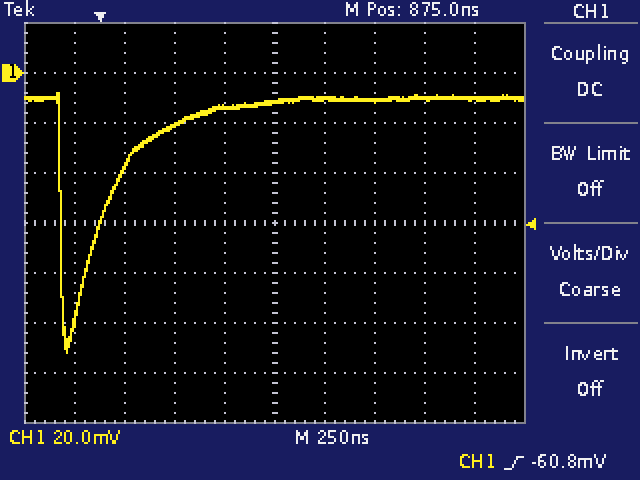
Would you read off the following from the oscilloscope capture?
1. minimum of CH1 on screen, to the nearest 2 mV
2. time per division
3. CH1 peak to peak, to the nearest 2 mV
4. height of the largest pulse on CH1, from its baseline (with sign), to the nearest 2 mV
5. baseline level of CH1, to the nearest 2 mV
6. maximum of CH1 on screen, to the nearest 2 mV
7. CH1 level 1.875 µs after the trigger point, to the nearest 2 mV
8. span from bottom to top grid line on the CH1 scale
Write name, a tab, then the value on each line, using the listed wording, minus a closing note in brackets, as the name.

minimum of CH1 on screen, to the nearest 2 mV	-112 mV
time per division	250 ns
CH1 peak to peak, to the nearest 2 mV	104 mV
height of the largest pulse on CH1, from its baseline (with sign), to the nearest 2 mV	-102 mV
baseline level of CH1, to the nearest 2 mV	-10 mV
maximum of CH1 on screen, to the nearest 2 mV	-8 mV
CH1 level 1.875 µs after the trigger point, to the nearest 2 mV	-10 mV
span from bottom to top grid line on the CH1 scale	160 mV
